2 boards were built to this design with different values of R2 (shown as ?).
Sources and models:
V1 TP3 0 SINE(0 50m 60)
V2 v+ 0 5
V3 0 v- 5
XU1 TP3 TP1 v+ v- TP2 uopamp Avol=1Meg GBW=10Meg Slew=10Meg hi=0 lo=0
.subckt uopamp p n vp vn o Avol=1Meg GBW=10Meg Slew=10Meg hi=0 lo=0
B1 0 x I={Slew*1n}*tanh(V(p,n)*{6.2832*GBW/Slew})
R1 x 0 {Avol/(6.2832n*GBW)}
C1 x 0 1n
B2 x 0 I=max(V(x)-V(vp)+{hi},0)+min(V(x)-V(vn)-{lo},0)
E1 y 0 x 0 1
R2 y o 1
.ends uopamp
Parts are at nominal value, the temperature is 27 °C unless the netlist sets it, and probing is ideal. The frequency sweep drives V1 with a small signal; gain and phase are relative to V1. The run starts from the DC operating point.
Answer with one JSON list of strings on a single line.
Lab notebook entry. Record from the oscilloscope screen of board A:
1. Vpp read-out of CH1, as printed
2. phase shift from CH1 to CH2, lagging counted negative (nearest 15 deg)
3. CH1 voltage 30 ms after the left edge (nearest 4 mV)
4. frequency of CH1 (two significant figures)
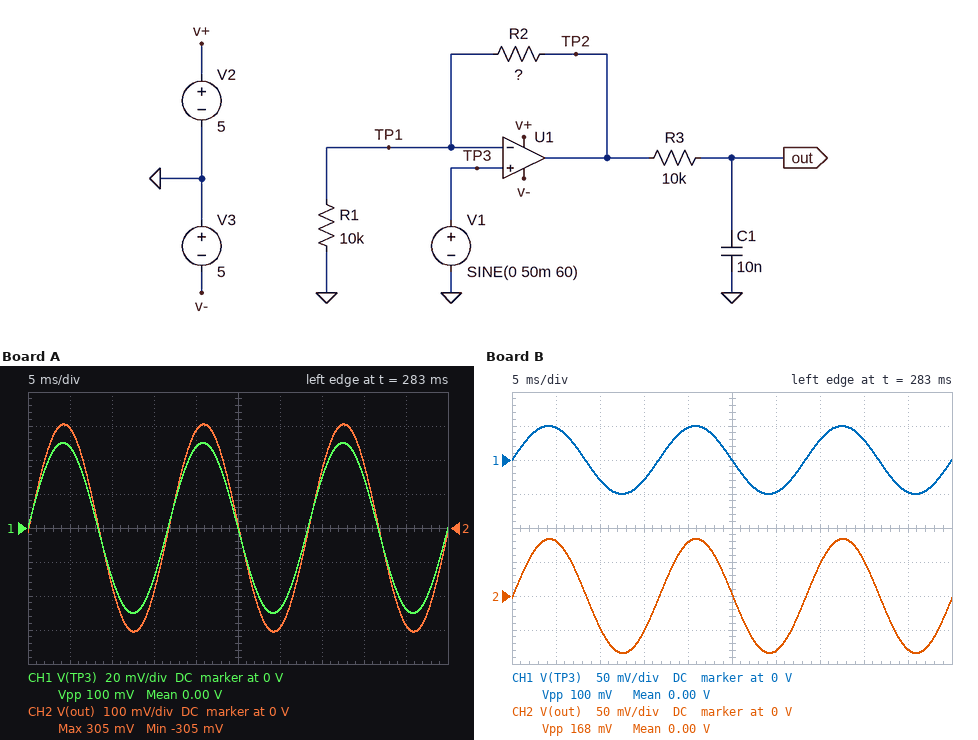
["100 mV", "0 deg", "-48 mV", "60 Hz"]
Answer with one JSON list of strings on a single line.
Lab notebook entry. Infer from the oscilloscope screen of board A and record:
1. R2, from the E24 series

["51 kΩ"]
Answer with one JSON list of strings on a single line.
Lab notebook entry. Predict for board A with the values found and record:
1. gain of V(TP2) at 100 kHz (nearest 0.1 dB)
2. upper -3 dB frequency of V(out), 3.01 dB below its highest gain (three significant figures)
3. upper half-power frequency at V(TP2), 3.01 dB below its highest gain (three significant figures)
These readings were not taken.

["15.7 dB", "1.59 kHz", "1.64 MHz"]
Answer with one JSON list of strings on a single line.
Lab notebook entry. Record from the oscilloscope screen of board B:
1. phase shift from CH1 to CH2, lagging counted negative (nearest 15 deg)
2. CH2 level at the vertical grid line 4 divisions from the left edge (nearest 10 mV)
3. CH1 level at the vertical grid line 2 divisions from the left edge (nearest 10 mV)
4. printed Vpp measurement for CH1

["0 deg", "80 mV", "-30 mV", "100 mV"]
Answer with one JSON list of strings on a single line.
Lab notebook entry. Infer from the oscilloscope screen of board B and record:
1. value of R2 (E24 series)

["6.8 kΩ"]
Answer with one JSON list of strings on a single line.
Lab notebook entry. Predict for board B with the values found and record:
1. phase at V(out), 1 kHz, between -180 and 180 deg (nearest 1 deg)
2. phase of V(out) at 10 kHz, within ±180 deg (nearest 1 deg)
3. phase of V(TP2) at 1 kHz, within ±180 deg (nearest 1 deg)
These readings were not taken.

["-32 deg", "-81 deg", "0 deg"]
